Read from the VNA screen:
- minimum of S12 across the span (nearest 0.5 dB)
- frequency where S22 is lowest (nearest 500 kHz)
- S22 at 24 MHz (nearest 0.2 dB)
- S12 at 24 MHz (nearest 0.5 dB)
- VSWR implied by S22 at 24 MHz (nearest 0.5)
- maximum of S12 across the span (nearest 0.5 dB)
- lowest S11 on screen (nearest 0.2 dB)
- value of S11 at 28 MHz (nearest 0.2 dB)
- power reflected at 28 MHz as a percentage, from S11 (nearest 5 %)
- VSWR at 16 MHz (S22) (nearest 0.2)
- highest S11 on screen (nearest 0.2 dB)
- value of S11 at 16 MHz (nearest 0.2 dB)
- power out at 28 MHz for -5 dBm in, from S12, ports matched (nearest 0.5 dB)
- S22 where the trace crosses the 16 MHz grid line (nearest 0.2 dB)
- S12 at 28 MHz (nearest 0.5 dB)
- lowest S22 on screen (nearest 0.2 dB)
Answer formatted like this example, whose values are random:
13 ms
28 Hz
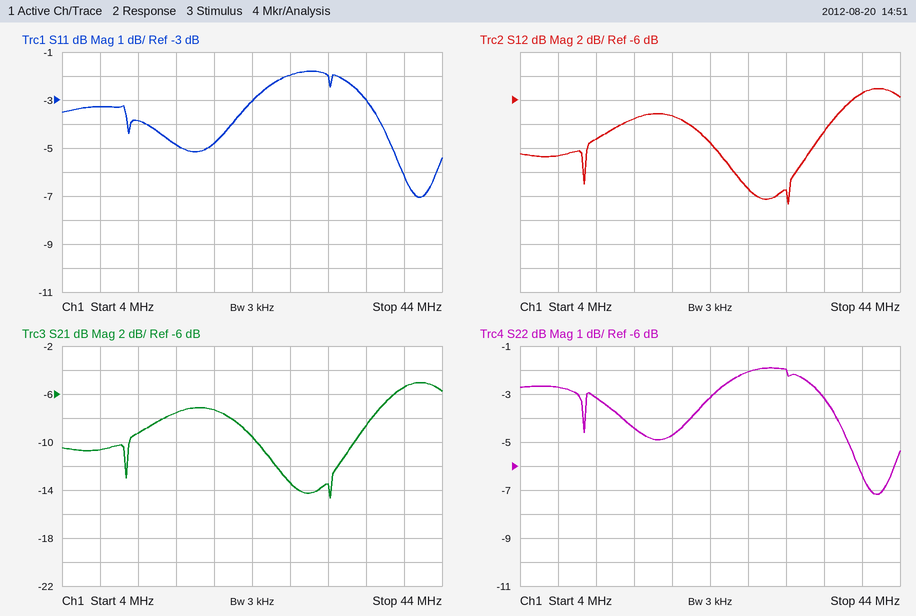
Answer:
-14.5 dB
41.5 MHz
-3.2 dB
-9.5 dB
5.5
-5.0 dB
-7.0 dB
-2.0 dB
65 %
4.0
-1.8 dB
-4.8 dB
-18.5 dBm
-4.4 dB
-13.5 dB
-7.2 dB
